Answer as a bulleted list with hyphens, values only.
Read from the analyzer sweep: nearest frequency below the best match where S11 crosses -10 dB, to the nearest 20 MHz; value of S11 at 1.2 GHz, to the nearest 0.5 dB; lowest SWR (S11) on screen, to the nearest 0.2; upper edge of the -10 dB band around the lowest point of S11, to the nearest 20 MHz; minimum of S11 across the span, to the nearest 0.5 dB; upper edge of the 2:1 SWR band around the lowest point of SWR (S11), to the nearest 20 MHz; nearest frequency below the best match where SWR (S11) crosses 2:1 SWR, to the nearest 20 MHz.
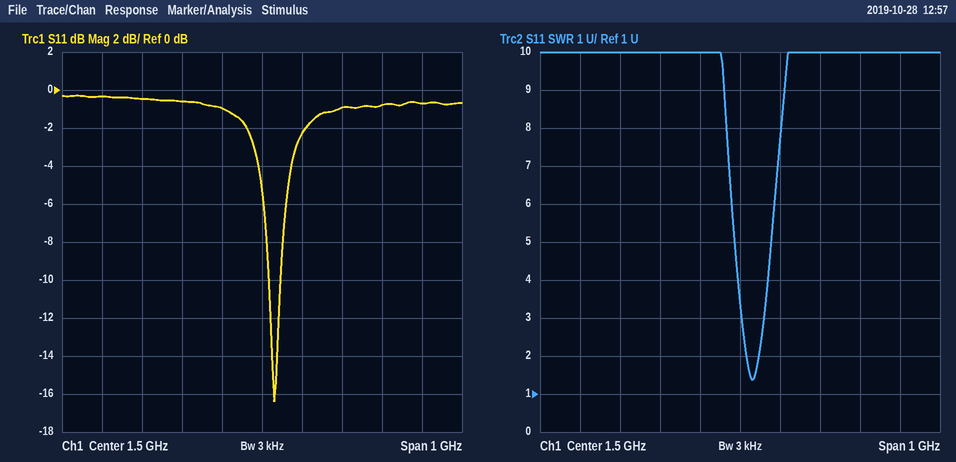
- 1.52 GHz
- -0.5 dB
- 1.4
- 1.54 GHz
- -16.5 dB
- 1.54 GHz
- 1.52 GHz
